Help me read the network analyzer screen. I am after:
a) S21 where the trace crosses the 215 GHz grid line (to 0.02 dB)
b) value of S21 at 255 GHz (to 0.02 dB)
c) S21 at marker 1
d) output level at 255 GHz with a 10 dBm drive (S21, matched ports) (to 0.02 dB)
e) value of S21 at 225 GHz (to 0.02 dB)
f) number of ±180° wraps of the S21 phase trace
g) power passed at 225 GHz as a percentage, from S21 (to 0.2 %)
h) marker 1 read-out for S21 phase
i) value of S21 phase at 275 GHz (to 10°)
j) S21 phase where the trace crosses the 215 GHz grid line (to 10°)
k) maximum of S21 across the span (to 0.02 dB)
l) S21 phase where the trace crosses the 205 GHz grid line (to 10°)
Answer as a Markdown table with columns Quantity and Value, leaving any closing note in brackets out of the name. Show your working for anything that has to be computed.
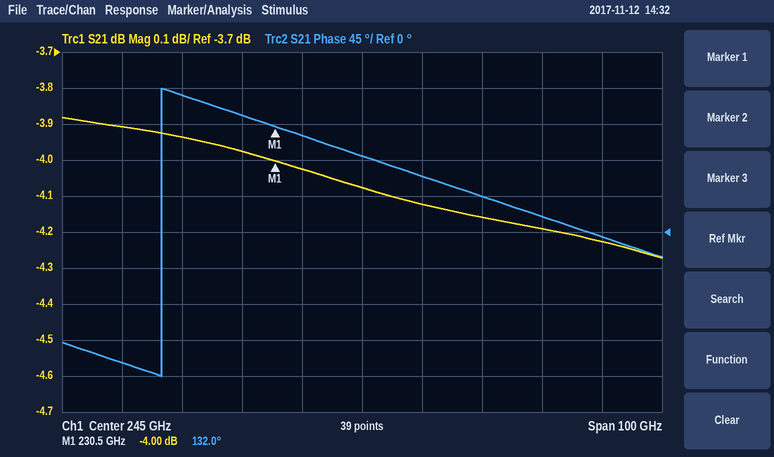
| Quantity | Value |
|---|---|
| S21 where the trace crosses the 215 GHz grid line | -3.94 dB |
| value of S21 at 255 GHz | -4.12 dB |
| S21 at marker 1 | -4.00 dB |
| output level at 255 GHz with a 10 dBm drive (S21, matched ports) | 10 dBm + (-4.12 dB) = 5.88 dBm |
| value of S21 at 225 GHz | -3.98 dB |
| number of ±180° wraps of the S21 phase trace | 1 |
| power passed at 225 GHz as a percentage, from S21 | 10^(-3.98/10) ≈ 40.0 % |
| marker 1 read-out for S21 phase | 132.0° |
| value of S21 phase at 275 GHz | 20° |
| S21 phase where the trace crosses the 215 GHz grid line | 170° |
| maximum of S21 across the span | -3.88 dB |
| S21 phase where the trace crosses the 205 GHz grid line | -160° |
